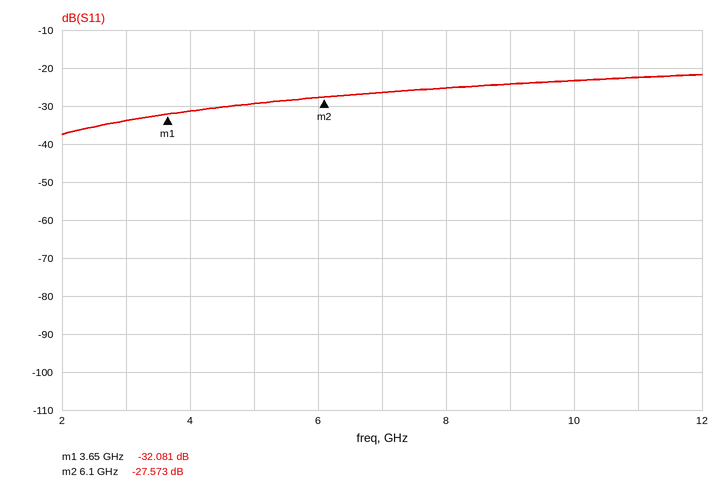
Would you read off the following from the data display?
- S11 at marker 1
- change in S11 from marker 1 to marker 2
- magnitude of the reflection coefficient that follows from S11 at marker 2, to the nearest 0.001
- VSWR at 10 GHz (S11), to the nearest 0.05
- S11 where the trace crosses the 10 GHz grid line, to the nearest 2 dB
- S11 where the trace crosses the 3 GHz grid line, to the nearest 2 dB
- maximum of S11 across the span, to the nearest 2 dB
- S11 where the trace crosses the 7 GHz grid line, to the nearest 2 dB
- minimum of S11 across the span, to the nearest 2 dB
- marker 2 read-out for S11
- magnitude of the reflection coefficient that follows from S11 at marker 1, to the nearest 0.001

-32.081 dB
4.508 dB
0.042
1.15
-24 dB
-34 dB
-22 dB
-26 dB
-38 dB
-27.573 dB
0.025
